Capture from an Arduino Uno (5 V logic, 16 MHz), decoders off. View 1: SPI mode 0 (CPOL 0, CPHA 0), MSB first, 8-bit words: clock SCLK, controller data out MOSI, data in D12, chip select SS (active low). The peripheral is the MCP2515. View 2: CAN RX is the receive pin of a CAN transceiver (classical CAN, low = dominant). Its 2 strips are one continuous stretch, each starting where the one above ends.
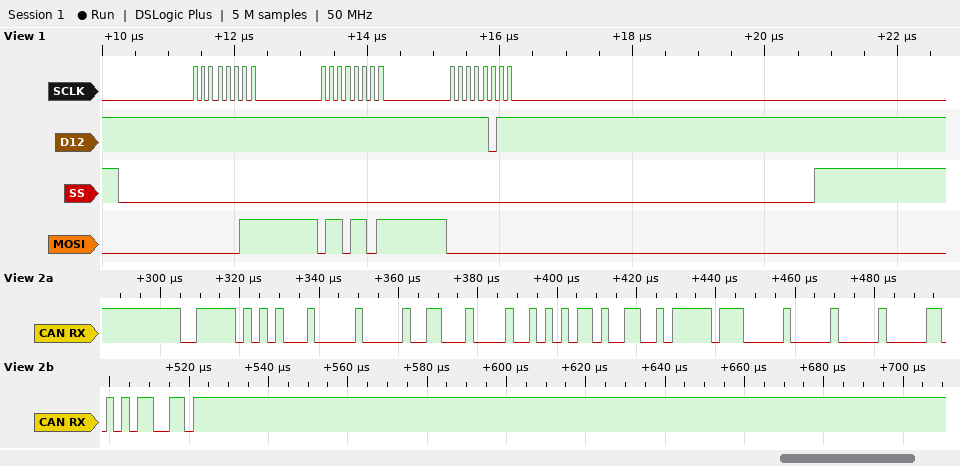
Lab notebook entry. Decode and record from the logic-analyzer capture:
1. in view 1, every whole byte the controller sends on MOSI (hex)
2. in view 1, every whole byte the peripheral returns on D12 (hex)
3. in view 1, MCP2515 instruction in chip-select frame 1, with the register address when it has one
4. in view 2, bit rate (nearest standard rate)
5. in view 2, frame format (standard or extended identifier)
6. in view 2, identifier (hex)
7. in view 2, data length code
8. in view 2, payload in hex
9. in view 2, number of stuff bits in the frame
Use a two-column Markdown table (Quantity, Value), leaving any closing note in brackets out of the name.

| Quantity | Value |
|---|---|
| in view 1, every whole byte the controller sends on MOSI | 03 6D 00 |
| in view 1, every whole byte the peripheral returns on D12 | FF FF FB |
| in view 1, MCP2515 instruction in chip-select frame 1, with the register address when it has one | READ 0x6D |
| in view 2, bit rate | 500 kbit/s |
| in view 2, frame format | standard |
| in view 2, identifier | 0x3F5 |
| in view 2, data length code | 8 |
| in view 2, payload in hex | 00 62 12 AD 32 FF 00 00 |
| in view 2, number of stuff bits in the frame | 8 |
